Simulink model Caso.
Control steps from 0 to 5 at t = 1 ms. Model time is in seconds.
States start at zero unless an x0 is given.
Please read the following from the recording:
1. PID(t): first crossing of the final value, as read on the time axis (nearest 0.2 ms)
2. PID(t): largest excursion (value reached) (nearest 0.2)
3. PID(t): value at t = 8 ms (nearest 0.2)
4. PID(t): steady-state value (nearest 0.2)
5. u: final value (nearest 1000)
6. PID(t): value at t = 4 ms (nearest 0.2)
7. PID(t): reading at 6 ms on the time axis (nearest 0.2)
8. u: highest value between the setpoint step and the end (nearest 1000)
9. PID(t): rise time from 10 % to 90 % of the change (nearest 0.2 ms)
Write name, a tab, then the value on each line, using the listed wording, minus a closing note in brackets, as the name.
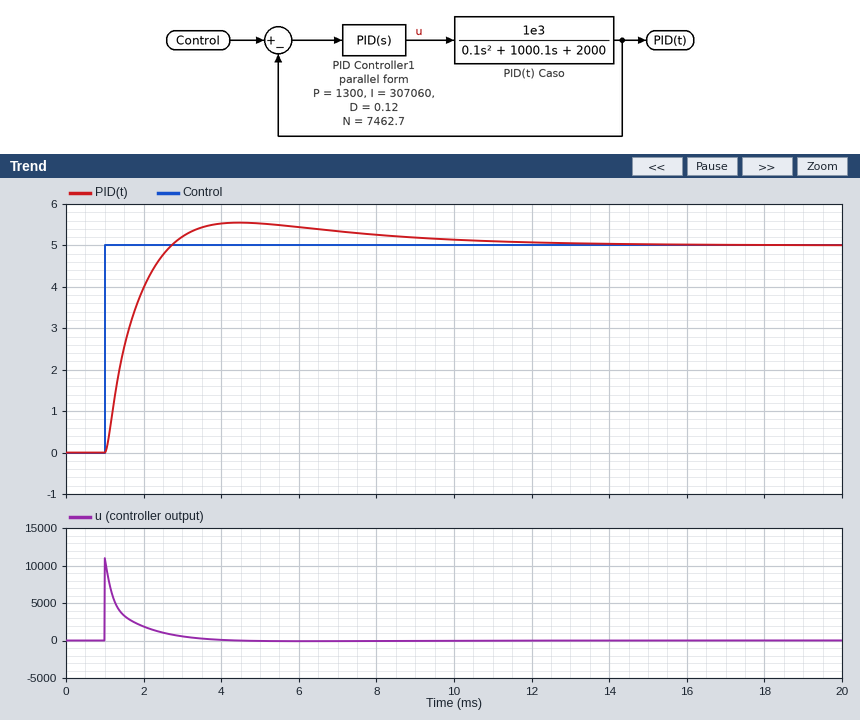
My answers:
PID(t): first crossing of the final value, as read on the time axis	2.8 ms
PID(t): largest excursion (value reached)	5.6
PID(t): value at t = 8 ms	5.2
PID(t): steady-state value	5.0
u: final value	0
PID(t): value at t = 4 ms	5.6
PID(t): reading at 6 ms on the time axis	5.4
u: highest value between the setpoint step and the end	11000
PID(t): rise time from 10 % to 90 % of the change	1.2 ms
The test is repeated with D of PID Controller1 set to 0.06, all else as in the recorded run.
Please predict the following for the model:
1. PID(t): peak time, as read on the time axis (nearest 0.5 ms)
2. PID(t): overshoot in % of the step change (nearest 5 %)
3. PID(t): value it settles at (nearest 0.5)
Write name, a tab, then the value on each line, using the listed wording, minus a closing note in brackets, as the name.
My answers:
PID(t): peak time, as read on the time axis	4.5 ms
PID(t): overshoot in % of the step change	10 %
PID(t): value it settles at	5.0
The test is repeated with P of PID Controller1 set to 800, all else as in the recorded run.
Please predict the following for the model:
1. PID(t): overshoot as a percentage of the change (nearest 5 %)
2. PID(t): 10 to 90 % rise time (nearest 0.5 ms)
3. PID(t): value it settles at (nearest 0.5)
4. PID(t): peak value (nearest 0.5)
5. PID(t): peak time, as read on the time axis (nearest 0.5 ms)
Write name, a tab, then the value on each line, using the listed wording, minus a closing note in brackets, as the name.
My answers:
PID(t): overshoot as a percentage of the change	20 %
PID(t): 10 to 90 % rise time	1.5 ms
PID(t): value it settles at	5.0
PID(t): peak value	6.0
PID(t): peak time, as read on the time axis	5.0 ms
